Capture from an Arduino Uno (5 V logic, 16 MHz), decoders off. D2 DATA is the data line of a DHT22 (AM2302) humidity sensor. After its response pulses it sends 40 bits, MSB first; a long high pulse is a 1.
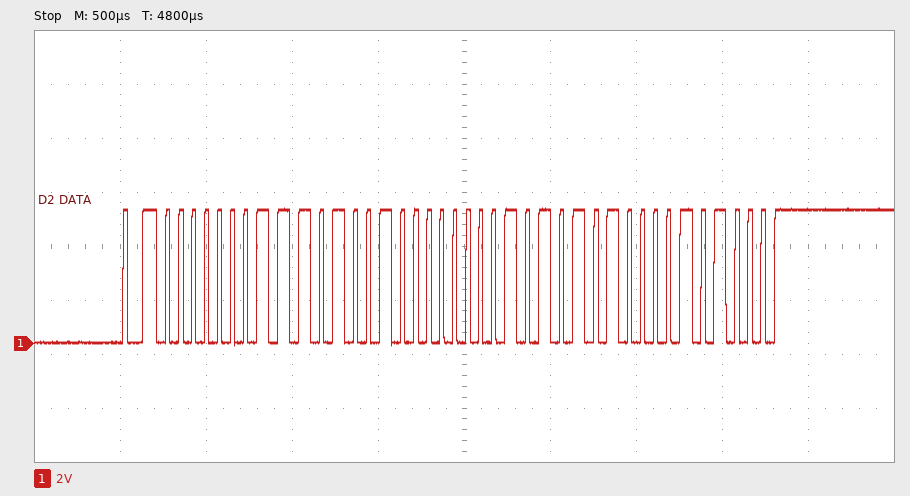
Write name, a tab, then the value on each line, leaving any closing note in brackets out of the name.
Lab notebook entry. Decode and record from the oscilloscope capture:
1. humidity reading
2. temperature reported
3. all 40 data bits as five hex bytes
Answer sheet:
humidity reading	46.6 %
temperature reported	34.0 °C
all 40 data bits as five hex bytes	01 D2 01 54 28
